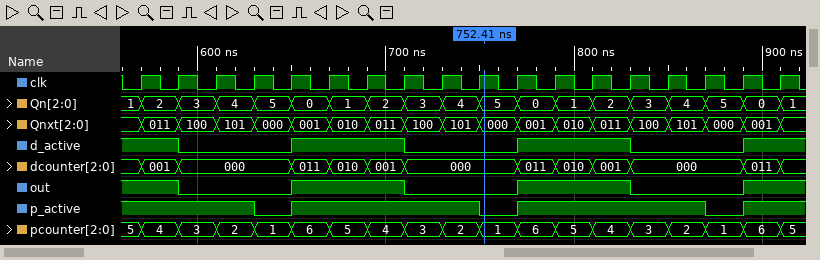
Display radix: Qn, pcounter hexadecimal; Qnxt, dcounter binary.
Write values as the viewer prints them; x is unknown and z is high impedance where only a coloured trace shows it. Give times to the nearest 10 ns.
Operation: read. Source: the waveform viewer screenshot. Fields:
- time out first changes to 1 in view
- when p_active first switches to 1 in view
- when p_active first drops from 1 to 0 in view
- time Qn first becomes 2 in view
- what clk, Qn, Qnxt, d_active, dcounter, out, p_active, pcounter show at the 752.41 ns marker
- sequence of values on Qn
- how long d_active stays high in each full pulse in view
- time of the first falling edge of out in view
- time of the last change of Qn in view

650 ns
650 ns
630 ns
570 ns
clk=1, Qn=5, Qnxt=000, d_active=0, dcounter=000, out=0, p_active=0, pcounter=1
1, 2, 3, 4, 5, 0, 1, 2, 3, 4, 5, 0, 1, 2, 3, 4, 5, 0, 1
60 ns, 60 ns
590 ns
910 ns
